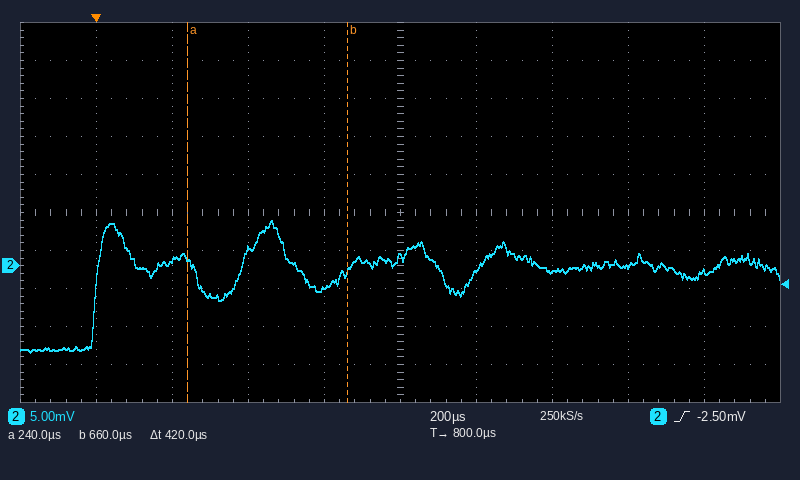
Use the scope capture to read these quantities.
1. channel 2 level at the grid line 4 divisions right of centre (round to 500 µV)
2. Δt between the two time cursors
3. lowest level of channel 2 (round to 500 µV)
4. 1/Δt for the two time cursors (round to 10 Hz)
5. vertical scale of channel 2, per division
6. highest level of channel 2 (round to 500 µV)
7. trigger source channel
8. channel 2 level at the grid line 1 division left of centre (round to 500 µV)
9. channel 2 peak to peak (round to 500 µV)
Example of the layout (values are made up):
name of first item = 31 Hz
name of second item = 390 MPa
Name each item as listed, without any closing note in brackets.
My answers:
channel 2 level at the grid line 4 divisions right of centre = -1.0 mV
Δt between the two time cursors = 420 µs
lowest level of channel 2 = -11.5 mV
1/Δt for the two time cursors = 2.38 kHz
vertical scale of channel 2, per division = 5 mV
highest level of channel 2 = 6.0 mV
trigger source channel = channel 2
channel 2 level at the grid line 1 division left of centre = -3.0 mV
channel 2 peak to peak = 17.5 mV
